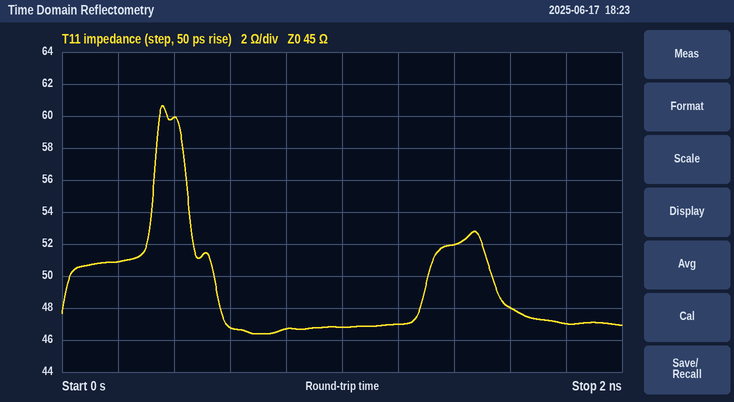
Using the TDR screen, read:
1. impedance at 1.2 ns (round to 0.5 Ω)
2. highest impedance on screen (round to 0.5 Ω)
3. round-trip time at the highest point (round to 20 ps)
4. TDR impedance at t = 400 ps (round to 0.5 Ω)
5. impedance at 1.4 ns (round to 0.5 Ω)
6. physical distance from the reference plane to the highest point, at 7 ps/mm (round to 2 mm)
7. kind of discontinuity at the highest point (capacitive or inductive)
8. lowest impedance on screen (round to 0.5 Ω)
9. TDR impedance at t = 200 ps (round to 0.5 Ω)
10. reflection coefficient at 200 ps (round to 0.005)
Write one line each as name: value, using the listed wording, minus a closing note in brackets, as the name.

impedance at 1.2 ns: 47.0 Ω
highest impedance on screen: 60.5 Ω
round-trip time at the highest point: 360 ps
TDR impedance at t = 400 ps: 60.0 Ω
impedance at 1.4 ns: 52.0 Ω
physical distance from the reference plane to the highest point, at 7 ps/mm: 26 mm
kind of discontinuity at the highest point: inductive
lowest impedance on screen: 46.5 Ω
TDR impedance at t = 200 ps: 51.0 Ω
reflection coefficient at 200 ps: +0.060
